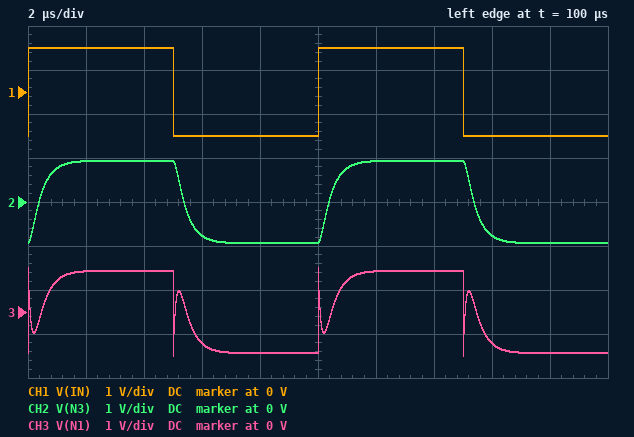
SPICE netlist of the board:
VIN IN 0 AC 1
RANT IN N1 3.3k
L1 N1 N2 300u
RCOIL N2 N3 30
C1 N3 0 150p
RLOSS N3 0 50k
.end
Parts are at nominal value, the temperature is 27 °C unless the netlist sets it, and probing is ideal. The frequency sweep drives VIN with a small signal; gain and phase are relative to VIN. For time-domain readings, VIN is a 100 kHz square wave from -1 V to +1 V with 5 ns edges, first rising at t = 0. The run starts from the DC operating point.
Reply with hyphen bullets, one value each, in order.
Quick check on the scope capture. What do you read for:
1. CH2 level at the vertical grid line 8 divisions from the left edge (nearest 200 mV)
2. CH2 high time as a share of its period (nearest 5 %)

- -800 mV
- 50 %
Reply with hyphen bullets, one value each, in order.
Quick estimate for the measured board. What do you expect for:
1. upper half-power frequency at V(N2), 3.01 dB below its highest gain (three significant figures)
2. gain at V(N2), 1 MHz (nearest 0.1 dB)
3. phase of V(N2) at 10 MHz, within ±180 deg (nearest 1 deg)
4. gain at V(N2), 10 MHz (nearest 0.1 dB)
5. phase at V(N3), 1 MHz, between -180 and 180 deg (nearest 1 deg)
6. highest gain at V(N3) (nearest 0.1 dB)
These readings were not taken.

- 408 kHz
- -10.2 dB
- -154 deg
- -44.7 dB
- -103 deg
- -0.6 dB
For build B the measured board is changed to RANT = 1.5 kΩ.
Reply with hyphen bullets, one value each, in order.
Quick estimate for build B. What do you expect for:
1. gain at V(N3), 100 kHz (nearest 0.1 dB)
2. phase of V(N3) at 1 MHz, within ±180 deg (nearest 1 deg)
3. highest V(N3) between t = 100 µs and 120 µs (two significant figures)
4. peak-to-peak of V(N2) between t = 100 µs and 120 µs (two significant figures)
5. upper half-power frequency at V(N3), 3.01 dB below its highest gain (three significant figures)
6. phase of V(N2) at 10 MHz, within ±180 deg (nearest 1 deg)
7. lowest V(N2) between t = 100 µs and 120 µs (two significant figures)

- -0.2 dB
- -117 deg
- 1.2 V
- 2.4 V
- 874 kHz
- -159 deg
- -1.2 V
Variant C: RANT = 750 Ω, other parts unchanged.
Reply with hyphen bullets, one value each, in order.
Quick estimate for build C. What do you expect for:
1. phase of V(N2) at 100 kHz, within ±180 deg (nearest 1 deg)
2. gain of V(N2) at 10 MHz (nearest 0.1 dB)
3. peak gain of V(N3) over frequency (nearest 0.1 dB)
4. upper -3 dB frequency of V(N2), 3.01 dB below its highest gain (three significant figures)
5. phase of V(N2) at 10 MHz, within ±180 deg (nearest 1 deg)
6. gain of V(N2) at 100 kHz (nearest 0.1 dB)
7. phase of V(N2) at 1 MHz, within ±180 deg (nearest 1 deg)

- -4 deg
- -44.6 dB
- 5.0 dB
- 890 kHz
- -162 deg
- 0 dB
- -133 deg
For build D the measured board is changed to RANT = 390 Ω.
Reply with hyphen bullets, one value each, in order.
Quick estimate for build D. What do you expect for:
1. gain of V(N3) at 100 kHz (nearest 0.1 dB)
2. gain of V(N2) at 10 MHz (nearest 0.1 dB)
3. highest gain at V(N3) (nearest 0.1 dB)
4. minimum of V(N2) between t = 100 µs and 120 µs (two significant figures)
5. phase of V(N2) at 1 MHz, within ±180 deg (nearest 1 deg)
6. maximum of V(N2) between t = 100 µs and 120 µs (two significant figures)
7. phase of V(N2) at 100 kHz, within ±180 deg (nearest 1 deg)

- 0.1 dB
- -44.6 dB
- 9.8 dB
- -2.2 V
- -149 deg
- 2.2 V
- -2 deg
